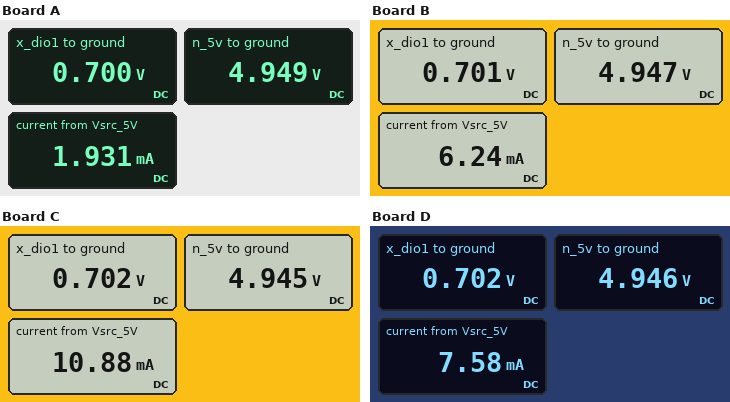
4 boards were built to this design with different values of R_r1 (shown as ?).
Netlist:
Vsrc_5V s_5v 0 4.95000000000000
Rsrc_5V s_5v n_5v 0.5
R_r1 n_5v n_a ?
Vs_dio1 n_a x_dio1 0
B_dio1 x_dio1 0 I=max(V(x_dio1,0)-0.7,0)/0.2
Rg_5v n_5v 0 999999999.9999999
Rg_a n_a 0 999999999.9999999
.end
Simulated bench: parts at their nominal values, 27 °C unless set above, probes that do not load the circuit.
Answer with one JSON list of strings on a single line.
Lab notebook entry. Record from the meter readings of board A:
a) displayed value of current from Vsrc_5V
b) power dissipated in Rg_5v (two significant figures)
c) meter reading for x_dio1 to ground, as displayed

["1.931 mA", "24 nW", "0.700 V"]
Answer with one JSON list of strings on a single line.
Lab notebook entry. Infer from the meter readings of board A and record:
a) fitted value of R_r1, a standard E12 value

["2.2 kΩ"]
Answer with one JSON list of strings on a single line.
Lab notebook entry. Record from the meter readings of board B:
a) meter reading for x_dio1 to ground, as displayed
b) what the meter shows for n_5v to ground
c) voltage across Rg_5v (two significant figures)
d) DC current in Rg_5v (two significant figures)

["0.701 V", "4.947 V", "4.9 V", "4.9 nA"]
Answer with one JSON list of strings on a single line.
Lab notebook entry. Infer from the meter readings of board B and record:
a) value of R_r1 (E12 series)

["680 Ω"]
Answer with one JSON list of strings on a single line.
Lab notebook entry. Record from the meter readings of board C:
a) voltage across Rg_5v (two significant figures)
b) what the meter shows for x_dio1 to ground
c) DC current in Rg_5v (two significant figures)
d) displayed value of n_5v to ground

["4.9 V", "0.702 V", "4.9 nA", "4.945 V"]
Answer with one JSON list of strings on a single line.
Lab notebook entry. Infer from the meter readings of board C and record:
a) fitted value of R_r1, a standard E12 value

["390 Ω"]
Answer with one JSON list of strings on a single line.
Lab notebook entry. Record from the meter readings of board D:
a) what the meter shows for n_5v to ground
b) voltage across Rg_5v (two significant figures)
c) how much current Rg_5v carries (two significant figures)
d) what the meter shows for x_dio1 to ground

["4.946 V", "4.9 V", "4.9 nA", "0.702 V"]
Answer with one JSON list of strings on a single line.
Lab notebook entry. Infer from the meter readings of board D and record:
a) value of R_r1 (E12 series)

["560 Ω"]
